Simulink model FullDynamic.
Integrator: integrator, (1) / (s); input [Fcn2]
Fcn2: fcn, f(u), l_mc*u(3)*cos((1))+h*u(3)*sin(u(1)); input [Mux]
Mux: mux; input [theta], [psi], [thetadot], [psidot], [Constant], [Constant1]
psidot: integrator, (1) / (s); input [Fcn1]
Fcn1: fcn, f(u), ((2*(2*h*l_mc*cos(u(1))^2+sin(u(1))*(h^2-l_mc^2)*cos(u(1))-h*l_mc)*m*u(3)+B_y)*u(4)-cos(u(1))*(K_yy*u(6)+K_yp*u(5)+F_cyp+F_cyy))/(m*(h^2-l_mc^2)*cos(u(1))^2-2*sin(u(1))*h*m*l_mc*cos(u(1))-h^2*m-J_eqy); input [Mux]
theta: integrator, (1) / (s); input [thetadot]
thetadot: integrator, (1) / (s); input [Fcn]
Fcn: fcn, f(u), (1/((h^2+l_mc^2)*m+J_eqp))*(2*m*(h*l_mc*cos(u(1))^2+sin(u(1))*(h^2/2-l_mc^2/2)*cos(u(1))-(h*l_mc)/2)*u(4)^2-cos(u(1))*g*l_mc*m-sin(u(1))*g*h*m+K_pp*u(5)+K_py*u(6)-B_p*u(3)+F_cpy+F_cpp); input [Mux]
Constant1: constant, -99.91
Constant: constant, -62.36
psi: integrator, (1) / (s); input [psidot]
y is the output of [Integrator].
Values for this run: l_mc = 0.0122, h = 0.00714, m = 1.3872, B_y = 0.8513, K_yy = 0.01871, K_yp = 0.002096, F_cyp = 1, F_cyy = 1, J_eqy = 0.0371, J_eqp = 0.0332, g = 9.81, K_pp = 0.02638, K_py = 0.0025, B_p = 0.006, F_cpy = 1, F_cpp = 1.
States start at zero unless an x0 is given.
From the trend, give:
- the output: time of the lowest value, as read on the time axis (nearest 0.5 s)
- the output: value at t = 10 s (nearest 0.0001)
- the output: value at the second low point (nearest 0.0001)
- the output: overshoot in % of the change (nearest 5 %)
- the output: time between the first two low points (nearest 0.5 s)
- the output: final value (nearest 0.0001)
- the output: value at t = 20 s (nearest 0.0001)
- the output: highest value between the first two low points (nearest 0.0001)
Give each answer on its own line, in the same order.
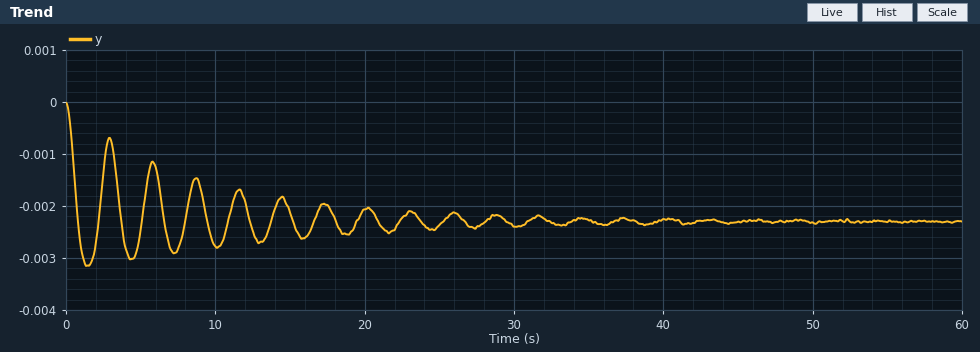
1.5 s
-0.0028
-0.0030
35 %
3.0 s
-0.0023
-0.0021
-0.0007
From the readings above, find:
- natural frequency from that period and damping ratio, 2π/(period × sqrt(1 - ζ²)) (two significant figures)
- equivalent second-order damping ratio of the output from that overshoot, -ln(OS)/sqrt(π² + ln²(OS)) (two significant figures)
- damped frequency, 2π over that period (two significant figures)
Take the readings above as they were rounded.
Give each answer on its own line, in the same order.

2.2 rad/s
0.32
2.1 rad/s
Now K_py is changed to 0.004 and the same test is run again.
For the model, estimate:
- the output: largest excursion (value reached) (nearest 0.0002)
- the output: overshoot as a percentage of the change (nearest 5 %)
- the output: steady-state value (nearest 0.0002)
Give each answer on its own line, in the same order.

-0.0036
10 %
-0.0034
